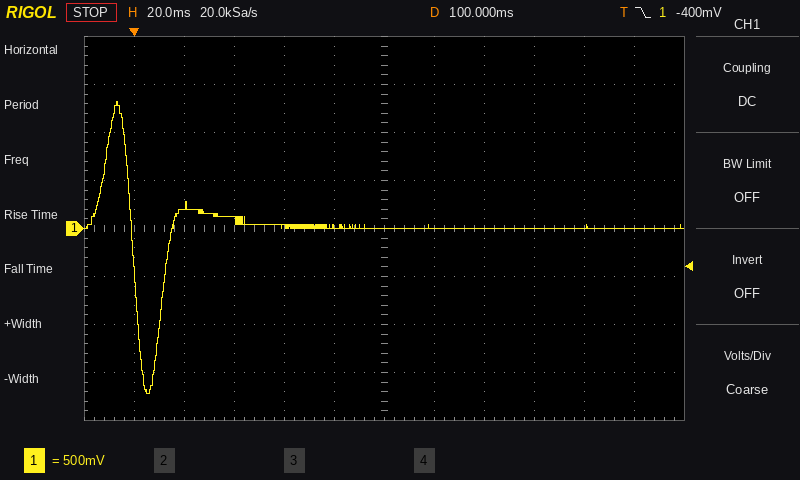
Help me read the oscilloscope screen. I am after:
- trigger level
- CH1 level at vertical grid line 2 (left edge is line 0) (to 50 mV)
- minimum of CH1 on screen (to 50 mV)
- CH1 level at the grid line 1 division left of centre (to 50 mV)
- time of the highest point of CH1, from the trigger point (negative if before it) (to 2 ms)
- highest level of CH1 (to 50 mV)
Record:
-400 mV
250 mV
-1.70 V
0 mV
-6 ms
1.30 V
